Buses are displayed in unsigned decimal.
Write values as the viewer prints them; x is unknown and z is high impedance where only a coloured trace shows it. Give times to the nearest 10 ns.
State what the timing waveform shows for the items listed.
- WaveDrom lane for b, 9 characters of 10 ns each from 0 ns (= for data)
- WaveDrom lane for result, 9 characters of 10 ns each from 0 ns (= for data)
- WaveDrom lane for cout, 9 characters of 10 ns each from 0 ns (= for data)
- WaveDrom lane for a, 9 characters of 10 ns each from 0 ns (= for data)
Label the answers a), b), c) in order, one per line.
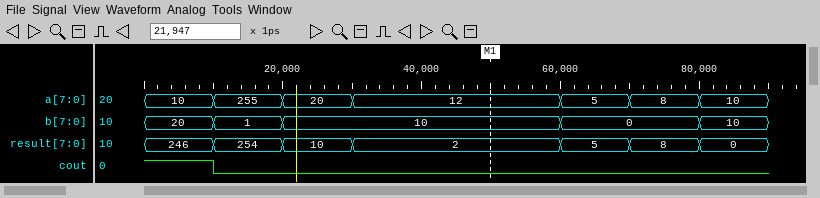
a) {name: 'b', wave: '===...=.=', data: '20 1 10 0 10'}
b) {name: 'result', wave: '====..===', data: '246 254 10 2 5 8 0'}
c) {name: 'cout', wave: '10.......'}
d) {name: 'a', wave: '====..===', data: '10 255 20 12 5 8 10'}
